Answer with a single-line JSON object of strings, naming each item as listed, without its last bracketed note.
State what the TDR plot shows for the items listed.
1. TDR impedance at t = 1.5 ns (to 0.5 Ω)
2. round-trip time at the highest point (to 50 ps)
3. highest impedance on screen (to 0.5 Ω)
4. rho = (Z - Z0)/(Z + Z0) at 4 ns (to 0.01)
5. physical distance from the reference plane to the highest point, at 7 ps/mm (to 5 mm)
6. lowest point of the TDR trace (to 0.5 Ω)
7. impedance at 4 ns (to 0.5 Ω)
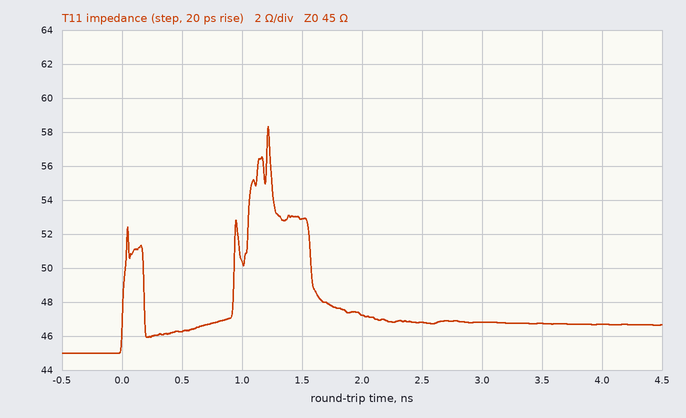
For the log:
{"TDR impedance at t = 1.5 ns": "53.0 Ω", "round-trip time at the highest point": "1.20 ns", "highest impedance on screen": "58.5 Ω", "rho = (Z - Z0)/(Z + Z0) at 4 ns": "+0.02", "physical distance from the reference plane to the highest point, at 7 ps/mm": "85 mm", "lowest point of the TDR trace": "45.0 Ω", "impedance at 4 ns": "46.5 Ω"}
